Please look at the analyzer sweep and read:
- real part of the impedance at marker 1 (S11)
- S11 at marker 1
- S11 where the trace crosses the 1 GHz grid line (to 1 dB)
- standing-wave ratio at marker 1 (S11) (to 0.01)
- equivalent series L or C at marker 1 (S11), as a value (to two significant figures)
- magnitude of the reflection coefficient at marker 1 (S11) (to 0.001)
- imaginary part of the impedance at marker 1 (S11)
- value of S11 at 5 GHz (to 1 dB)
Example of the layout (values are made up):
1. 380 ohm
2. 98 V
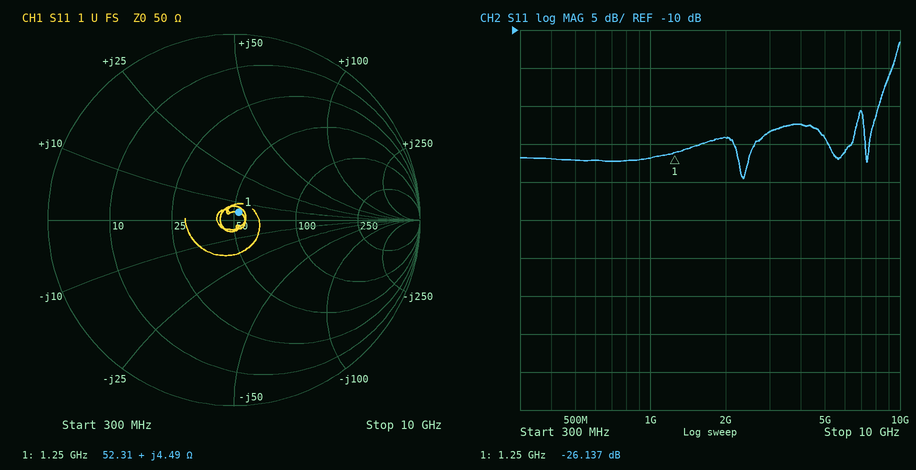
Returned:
1. 52.31 Ω
2. -26.137 dB
3. -27 dB
4. 1.10
5. 570 pH
6. 0.049
7. +4.49 Ω
8. -24 dB
